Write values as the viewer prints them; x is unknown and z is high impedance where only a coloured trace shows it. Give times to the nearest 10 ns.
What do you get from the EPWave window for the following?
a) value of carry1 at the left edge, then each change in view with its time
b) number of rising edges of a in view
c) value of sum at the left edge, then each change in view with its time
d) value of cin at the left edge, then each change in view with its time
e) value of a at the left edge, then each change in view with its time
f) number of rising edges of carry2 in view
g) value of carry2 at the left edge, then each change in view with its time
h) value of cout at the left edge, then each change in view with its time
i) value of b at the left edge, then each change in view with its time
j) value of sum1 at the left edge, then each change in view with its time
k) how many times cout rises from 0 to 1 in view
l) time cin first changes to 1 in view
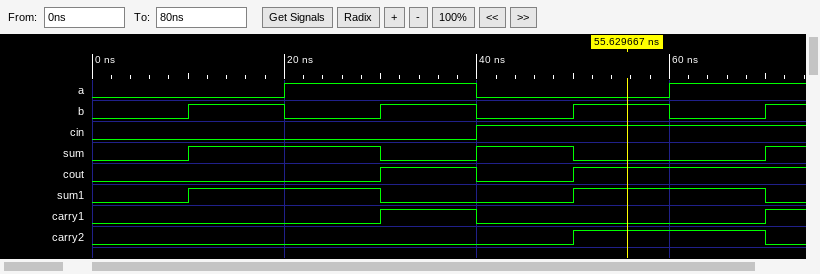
0, 1 at 30 ns, 0 at 40 ns, 1 at 70 ns
2
0, 1 at 10 ns, 0 at 30 ns, 1 at 40 ns, 0 at 50 ns, 1 at 70 ns
0, 1 at 40 ns
0, 1 at 20 ns, 0 at 40 ns, 1 at 60 ns
1
0, 1 at 50 ns, 0 at 70 ns
0, 1 at 30 ns, 0 at 40 ns, 1 at 50 ns
0, 1 at 10 ns, 0 at 20 ns, 1 at 30 ns, 0 at 40 ns, 1 at 50 ns, 0 at 60 ns, 1 at 70 ns
0, 1 at 10 ns, 0 at 30 ns, 1 at 50 ns, 0 at 70 ns
2
40 ns
